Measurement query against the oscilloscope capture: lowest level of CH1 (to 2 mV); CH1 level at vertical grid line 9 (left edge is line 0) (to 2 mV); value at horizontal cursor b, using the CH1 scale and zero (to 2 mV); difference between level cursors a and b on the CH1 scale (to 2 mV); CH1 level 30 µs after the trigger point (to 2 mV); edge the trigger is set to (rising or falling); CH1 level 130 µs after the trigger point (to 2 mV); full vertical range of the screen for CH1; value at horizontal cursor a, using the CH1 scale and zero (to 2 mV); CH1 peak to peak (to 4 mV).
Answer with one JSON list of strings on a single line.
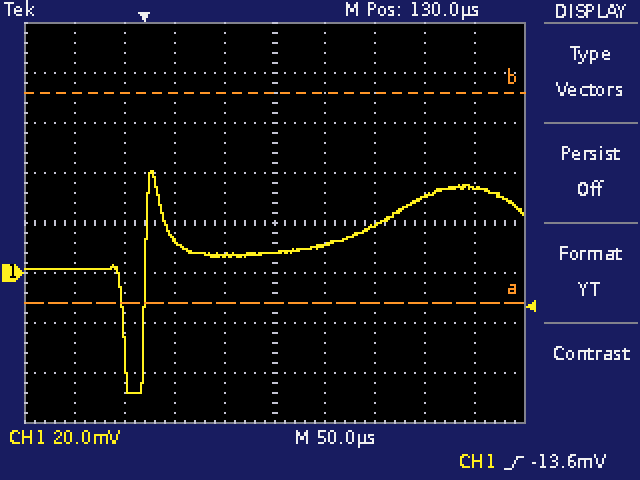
["-48 mV", "34 mV", "72 mV", "84 mV", "14 mV", "rising", "8 mV", "160 mV", "-12 mV", "88 mV"]
